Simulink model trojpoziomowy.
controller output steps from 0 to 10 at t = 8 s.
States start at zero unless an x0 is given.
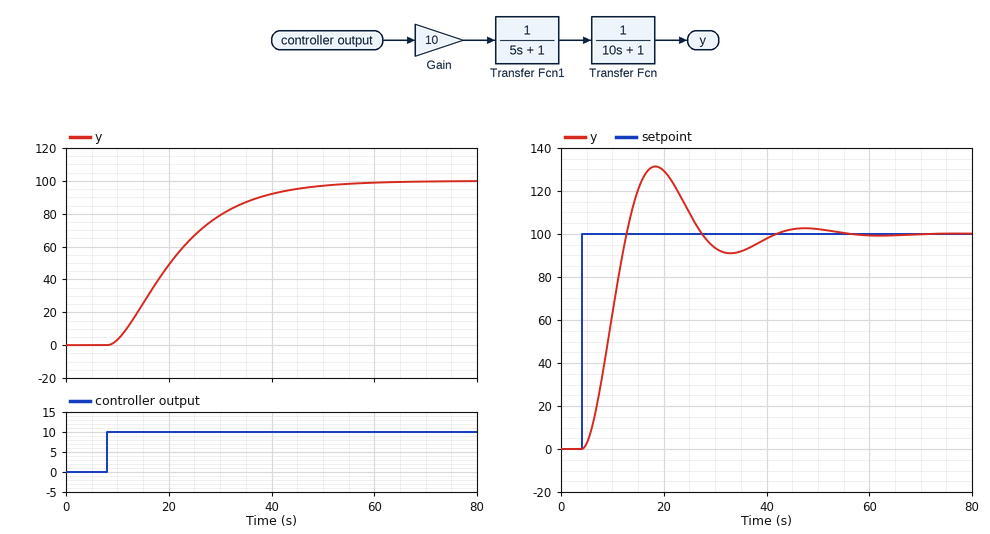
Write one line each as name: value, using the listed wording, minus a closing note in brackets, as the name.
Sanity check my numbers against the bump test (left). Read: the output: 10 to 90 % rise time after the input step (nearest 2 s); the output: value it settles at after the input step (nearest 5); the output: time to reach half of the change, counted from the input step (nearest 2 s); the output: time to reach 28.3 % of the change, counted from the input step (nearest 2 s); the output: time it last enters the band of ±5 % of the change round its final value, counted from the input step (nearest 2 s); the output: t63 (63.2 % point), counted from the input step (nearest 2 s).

the output: 10 to 90 % rise time after the input step: 26 s
the output: value it settles at after the input step: 100
the output: time to reach half of the change, counted from the input step: 12 s
the output: time to reach 28.3 % of the change, counted from the input step: 8 s
the output: time it last enters the band of ±5 % of the change round its final value, counted from the input step: 36 s
the output: t63 (63.2 % point), counted from the input step: 16 s
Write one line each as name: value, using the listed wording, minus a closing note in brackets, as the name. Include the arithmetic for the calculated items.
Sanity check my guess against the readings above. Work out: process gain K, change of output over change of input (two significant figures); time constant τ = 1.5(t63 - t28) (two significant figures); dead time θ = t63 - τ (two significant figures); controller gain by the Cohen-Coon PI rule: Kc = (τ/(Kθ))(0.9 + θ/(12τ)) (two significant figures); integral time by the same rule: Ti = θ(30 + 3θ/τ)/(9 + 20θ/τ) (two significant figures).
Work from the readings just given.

process gain K, change of output over change of input: (100 - 0) / 10 = 10
time constant τ = 1.5(t63 - t28): 1.5 × (16 - 8) = 12 s
dead time θ = t63 - τ: 16 - 12 = 4.0 s
controller gain by the Cohen-Coon PI rule: Kc = (τ/(Kθ))(0.9 + θ/(12τ)): 12 / (10 × 4) × (0.9 + 4 / (12 × 12)) = 0.28
integral time by the same rule: Ti = θ(30 + 3θ/τ)/(9 + 20θ/τ): 4 × (30 + 3 × 4 / 12) / (9 + 20 × 4 / 12) = 7.9 s
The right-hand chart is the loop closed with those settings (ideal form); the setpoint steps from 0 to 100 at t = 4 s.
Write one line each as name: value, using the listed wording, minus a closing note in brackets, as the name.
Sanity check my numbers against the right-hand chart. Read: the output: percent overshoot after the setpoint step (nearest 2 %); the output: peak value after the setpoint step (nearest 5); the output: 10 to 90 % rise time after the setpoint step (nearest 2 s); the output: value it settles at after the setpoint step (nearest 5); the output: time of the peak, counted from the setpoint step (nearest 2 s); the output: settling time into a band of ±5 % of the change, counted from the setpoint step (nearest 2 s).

the output: percent overshoot after the setpoint step: 32 %
the output: peak value after the setpoint step: 130
the output: 10 to 90 % rise time after the setpoint step: 6 s
the output: value it settles at after the setpoint step: 100
the output: time of the peak, counted from the setpoint step: 14 s
the output: settling time into a band of ±5 % of the change, counted from the setpoint step: 34 s
